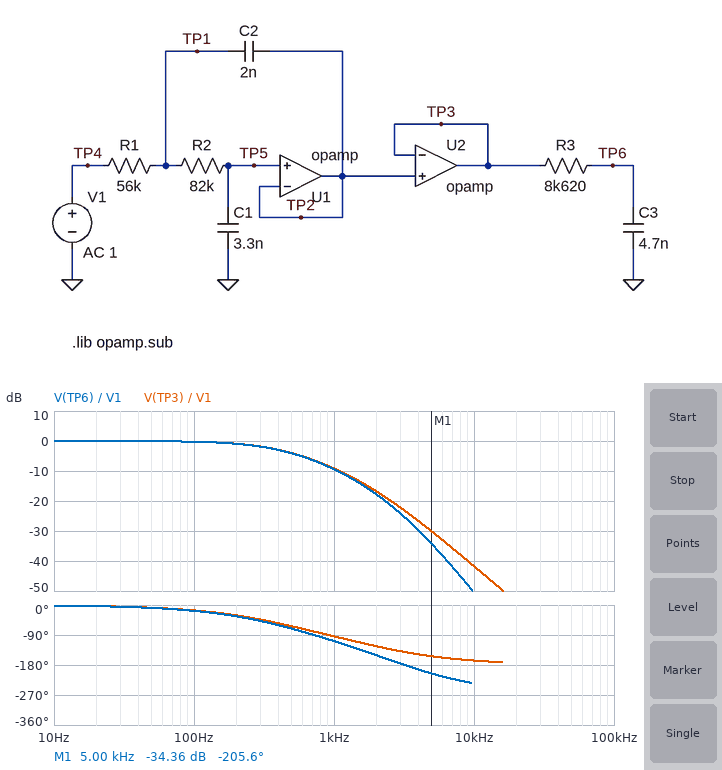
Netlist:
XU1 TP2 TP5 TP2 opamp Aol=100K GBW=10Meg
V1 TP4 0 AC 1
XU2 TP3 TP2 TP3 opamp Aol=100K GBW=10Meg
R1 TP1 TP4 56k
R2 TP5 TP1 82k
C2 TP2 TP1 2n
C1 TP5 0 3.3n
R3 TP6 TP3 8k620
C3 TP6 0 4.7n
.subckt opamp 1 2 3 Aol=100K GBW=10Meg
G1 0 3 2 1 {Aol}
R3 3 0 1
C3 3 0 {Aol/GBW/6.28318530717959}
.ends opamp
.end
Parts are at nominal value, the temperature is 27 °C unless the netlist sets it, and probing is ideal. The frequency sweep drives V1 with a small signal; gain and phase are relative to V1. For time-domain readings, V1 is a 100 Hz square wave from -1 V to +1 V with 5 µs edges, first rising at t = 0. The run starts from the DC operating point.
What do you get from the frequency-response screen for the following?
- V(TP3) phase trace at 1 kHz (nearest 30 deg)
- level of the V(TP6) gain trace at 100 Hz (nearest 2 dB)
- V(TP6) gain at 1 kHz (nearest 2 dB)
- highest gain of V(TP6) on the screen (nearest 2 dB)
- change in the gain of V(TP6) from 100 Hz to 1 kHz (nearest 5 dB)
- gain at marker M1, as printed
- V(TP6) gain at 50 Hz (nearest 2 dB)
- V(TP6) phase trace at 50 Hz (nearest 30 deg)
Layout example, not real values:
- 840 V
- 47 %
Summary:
- -90 deg
- 0 dB
- -10 dB
- 0 dB
- -10 dB
- -34.36 dB
- 0 dB
- 0 deg
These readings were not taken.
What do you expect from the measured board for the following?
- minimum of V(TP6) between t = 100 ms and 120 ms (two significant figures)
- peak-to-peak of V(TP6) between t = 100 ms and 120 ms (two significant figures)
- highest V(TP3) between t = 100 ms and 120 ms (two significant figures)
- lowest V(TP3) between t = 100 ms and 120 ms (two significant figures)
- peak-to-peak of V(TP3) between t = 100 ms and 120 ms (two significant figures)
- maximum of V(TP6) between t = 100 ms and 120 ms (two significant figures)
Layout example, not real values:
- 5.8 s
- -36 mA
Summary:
- -1.0 V
- 2.0 V
- 1.0 V
- -1.0 V
- 2.0 V
- 1.0 V
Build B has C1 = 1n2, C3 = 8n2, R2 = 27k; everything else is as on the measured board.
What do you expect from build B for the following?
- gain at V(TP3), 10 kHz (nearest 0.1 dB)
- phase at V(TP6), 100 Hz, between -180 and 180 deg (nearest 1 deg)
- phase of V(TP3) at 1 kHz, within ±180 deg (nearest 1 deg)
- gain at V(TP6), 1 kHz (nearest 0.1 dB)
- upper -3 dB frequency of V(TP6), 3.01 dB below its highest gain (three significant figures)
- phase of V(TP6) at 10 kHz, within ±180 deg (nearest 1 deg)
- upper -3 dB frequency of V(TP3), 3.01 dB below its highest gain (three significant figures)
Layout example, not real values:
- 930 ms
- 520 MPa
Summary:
- -23.4 dB
- -6 deg
- -36 deg
- -1.3 dB
- 1.54 kHz
- 128 deg
- 2.21 kHz
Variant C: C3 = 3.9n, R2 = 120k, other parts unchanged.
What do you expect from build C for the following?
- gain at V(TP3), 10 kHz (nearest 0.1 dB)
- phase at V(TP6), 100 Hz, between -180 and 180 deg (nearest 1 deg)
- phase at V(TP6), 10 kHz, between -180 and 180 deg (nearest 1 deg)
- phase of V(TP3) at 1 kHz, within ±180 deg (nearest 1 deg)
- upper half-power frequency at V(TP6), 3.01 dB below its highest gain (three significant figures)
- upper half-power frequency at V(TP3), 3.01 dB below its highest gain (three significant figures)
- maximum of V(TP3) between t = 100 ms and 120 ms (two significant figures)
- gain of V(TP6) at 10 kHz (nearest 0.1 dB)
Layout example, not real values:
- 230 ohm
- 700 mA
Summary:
- -45.0 dB
- -22 deg
- 127 deg
- -102 deg
- 313 Hz
- 314 Hz
- 1.0 V
- -52.4 dB
